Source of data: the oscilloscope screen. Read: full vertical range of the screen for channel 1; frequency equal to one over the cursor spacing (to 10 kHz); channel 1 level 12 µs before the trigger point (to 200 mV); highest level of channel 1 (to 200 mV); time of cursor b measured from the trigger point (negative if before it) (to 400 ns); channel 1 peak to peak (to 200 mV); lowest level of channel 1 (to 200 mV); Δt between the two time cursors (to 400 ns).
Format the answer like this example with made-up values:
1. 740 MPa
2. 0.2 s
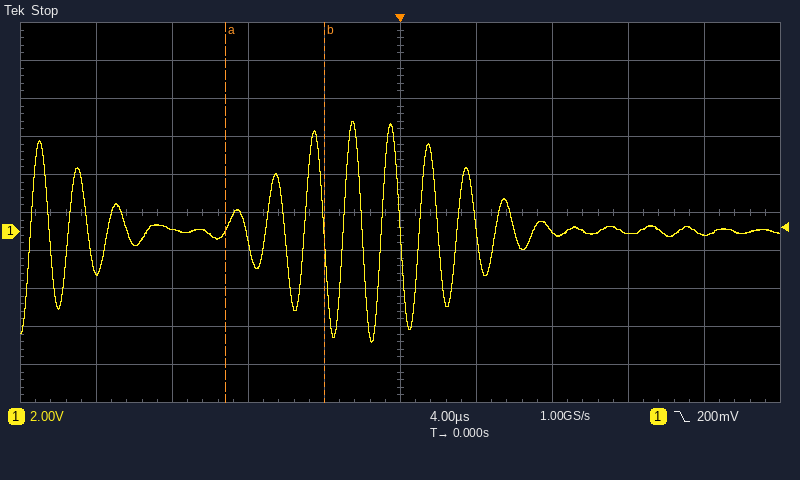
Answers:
1. 20 V
2. 190 kHz
3. 200 mV
4. 5.8 V
5. -4.0 µs
6. 11.6 V
7. -5.8 V
8. 5.2 µs
